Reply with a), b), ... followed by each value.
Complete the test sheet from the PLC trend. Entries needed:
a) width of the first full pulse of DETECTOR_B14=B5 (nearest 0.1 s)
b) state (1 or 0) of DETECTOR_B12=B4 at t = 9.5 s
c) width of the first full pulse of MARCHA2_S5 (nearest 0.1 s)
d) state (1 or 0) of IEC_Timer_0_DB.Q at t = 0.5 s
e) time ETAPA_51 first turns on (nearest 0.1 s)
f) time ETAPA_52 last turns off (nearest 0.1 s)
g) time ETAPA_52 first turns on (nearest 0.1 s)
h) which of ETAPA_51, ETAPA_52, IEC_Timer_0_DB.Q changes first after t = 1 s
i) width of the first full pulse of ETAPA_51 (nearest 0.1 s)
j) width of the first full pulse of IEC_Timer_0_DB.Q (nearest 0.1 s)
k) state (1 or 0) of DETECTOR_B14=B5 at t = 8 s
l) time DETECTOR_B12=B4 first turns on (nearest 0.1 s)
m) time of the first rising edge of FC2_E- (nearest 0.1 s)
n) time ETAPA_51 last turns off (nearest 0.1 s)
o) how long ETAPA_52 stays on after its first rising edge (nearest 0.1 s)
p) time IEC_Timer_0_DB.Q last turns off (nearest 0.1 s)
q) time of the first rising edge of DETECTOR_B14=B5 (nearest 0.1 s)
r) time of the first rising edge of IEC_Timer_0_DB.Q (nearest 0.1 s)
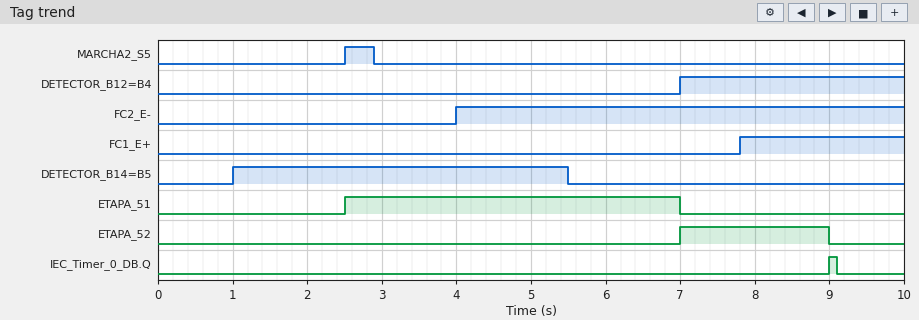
a) 4.5 s
b) 1
c) 0.4 s
d) 0
e) 2.5 s
f) 9.0 s
g) 7.0 s
h) ETAPA_51
i) 4.5 s
j) 0.1 s
k) 0
l) 7.0 s
m) 4.0 s
n) 7.0 s
o) 2.0 s
p) 9.1 s
q) 1.0 s
r) 9.0 s
